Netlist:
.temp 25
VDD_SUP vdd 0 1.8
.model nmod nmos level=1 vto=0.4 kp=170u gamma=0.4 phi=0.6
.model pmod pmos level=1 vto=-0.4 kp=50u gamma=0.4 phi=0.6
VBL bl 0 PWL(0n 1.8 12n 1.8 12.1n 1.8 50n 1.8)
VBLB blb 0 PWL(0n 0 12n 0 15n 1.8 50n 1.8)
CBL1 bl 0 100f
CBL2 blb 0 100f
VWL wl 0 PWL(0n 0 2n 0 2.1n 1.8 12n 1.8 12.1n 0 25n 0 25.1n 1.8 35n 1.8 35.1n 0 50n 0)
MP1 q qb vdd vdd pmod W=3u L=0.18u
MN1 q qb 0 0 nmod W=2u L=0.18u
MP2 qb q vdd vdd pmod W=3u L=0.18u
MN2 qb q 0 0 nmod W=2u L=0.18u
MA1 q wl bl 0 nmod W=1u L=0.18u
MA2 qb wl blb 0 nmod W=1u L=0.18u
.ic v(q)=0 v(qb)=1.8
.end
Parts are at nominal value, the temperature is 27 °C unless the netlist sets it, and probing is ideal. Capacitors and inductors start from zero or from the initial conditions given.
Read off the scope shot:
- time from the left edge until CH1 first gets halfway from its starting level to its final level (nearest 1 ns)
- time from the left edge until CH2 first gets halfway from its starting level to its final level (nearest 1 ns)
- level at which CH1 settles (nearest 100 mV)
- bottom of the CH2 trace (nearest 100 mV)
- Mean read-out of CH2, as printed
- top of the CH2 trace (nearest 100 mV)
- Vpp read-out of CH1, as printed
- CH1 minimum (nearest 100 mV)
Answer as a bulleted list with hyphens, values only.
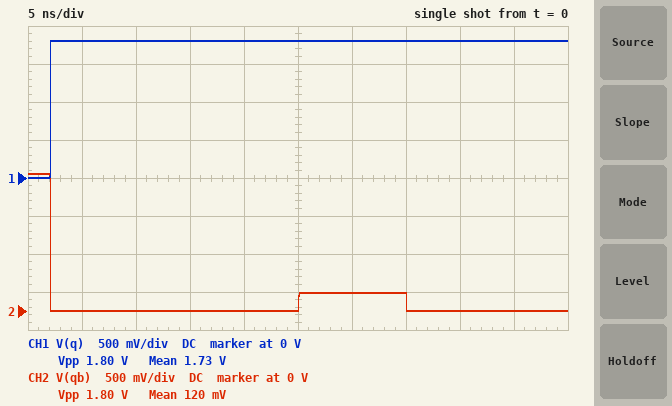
- 2 ns
- 2 ns
- 1.8 V
- 0 V
- 120 mV
- 1.8 V
- 1.80 V
- 0 V
